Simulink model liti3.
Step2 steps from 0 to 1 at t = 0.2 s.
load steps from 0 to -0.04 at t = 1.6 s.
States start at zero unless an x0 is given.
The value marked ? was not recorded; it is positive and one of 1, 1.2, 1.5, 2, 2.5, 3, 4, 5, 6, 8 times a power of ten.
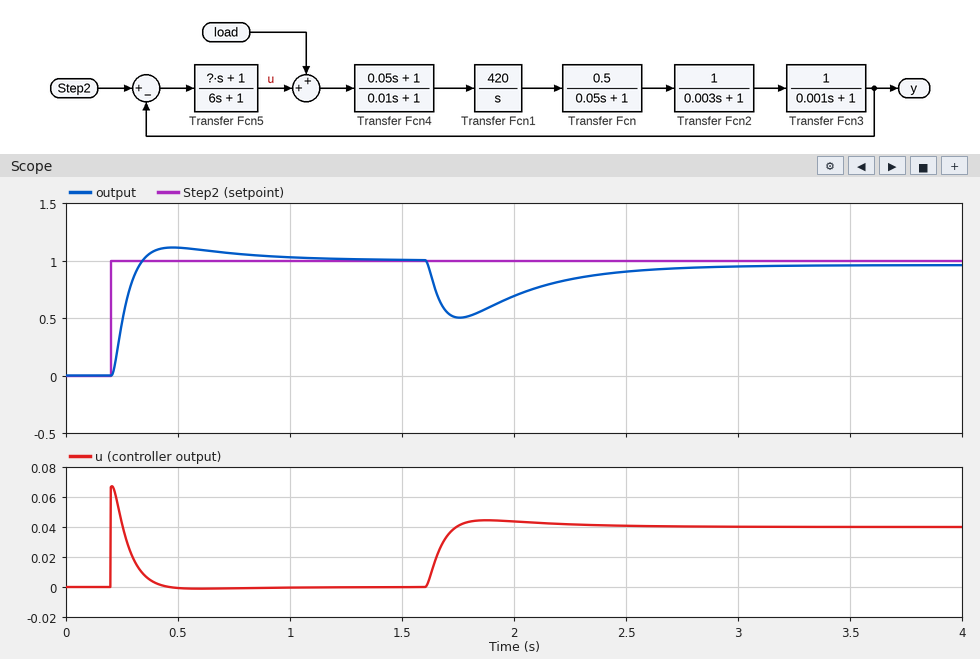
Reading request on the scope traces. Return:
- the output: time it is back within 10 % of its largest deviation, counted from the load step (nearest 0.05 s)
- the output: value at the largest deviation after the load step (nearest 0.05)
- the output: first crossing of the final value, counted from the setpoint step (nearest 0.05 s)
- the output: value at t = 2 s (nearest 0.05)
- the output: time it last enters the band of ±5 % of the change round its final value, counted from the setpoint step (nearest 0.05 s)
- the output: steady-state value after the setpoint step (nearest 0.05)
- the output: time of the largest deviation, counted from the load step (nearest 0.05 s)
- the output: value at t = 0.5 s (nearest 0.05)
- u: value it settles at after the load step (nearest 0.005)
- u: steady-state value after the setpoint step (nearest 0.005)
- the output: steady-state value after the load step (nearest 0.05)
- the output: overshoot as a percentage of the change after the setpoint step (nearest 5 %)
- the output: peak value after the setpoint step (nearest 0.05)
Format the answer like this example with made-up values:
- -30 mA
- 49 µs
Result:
- 0.95 s
- 0.50
- 0.15 s
- 0.70
- 0.60 s
- 1.00
- 0.15 s
- 1.10
- 0.040
- 0.000
- 0.95
- 10 %
- 1.10
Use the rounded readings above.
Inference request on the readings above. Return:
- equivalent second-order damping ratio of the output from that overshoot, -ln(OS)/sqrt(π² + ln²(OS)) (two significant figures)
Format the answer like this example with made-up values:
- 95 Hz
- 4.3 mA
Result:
- 0.59
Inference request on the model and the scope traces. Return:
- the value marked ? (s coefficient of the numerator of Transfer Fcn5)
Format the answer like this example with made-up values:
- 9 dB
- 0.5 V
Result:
- 0.4
